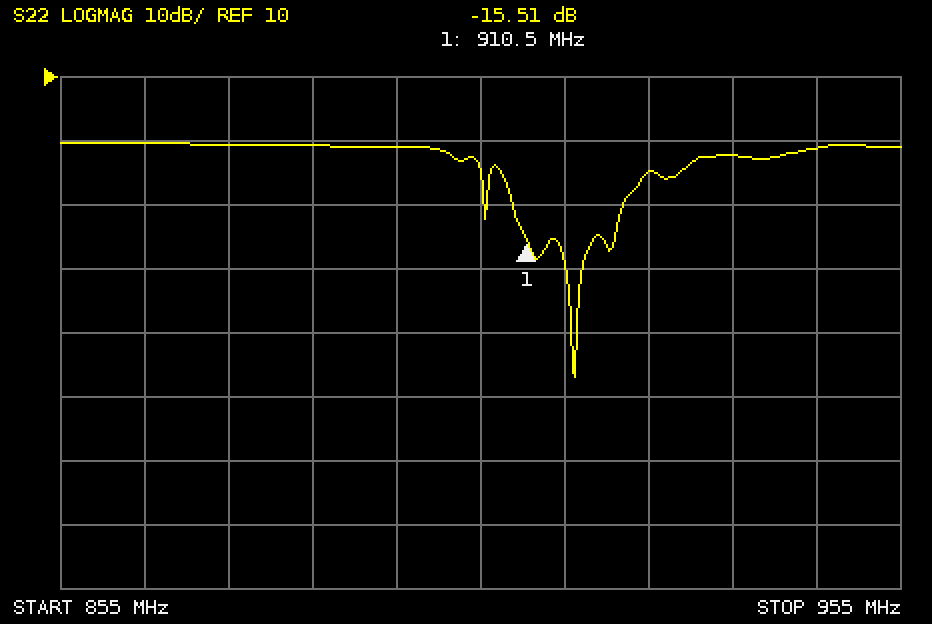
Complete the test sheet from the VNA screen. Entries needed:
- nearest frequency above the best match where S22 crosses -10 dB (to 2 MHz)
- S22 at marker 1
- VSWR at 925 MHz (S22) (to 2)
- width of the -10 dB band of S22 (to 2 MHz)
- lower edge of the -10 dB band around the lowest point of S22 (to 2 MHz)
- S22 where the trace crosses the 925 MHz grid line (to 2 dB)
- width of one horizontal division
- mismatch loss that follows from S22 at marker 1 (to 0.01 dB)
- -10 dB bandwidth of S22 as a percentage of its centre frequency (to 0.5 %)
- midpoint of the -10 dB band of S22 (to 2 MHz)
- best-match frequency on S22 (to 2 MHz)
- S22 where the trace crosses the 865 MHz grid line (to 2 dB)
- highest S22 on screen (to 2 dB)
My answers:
922 MHz
-15.51 dB
4
14 MHz
908 MHz
-4 dB
10 MHz
0.12 dB
1.5 %
916 MHz
916 MHz
0 dB
0 dB
